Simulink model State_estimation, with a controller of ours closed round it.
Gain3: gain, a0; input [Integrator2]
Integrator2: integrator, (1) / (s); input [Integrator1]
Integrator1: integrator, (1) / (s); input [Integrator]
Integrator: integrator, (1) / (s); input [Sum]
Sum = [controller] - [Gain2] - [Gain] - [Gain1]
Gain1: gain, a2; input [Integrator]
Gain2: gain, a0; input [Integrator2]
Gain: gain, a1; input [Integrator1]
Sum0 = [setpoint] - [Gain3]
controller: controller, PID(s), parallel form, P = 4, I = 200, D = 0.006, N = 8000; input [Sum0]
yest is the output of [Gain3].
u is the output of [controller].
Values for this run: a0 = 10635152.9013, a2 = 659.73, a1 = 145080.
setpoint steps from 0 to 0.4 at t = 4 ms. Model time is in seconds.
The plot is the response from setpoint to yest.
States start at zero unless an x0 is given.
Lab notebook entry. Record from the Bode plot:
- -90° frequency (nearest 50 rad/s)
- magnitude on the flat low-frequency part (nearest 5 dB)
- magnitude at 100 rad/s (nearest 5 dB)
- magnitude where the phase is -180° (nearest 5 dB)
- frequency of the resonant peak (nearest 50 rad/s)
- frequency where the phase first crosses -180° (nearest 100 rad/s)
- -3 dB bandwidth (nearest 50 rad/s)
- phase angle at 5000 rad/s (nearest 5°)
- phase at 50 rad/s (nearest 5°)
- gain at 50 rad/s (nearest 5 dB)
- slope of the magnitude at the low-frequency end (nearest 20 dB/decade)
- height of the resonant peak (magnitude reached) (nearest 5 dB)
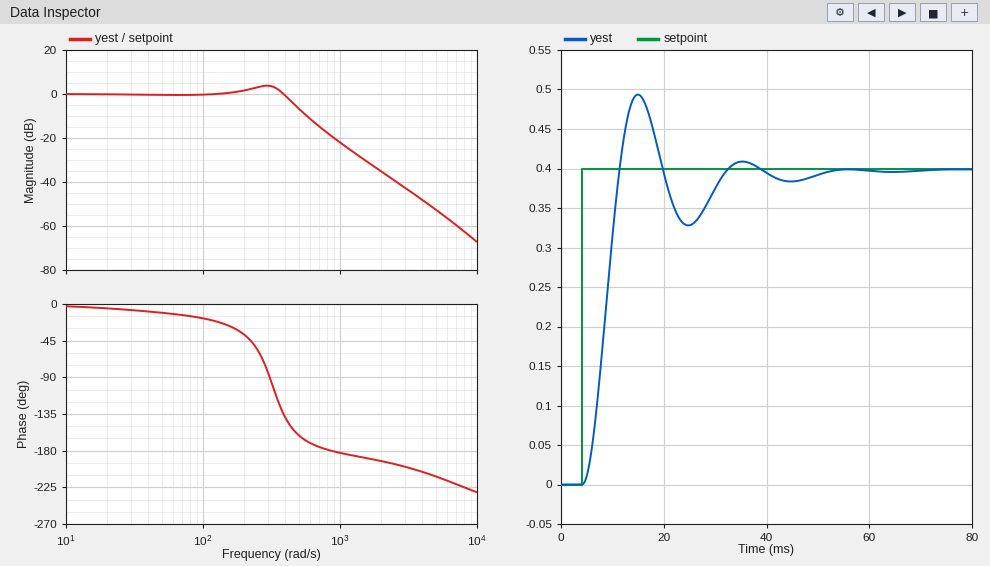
300 rad/s
0 dB
0 dB
-20 dB
300 rad/s
900 rad/s
450 rad/s
-210°
-10°
0 dB
0 dB/decade
5 dB
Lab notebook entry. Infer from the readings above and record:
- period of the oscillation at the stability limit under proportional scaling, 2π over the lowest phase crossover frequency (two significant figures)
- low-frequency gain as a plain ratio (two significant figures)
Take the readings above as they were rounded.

0.0070 s
1.0
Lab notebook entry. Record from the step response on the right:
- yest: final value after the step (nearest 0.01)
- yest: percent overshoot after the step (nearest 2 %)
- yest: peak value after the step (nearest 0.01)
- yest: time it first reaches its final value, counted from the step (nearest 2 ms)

0.40
24 %
0.49
8 ms
